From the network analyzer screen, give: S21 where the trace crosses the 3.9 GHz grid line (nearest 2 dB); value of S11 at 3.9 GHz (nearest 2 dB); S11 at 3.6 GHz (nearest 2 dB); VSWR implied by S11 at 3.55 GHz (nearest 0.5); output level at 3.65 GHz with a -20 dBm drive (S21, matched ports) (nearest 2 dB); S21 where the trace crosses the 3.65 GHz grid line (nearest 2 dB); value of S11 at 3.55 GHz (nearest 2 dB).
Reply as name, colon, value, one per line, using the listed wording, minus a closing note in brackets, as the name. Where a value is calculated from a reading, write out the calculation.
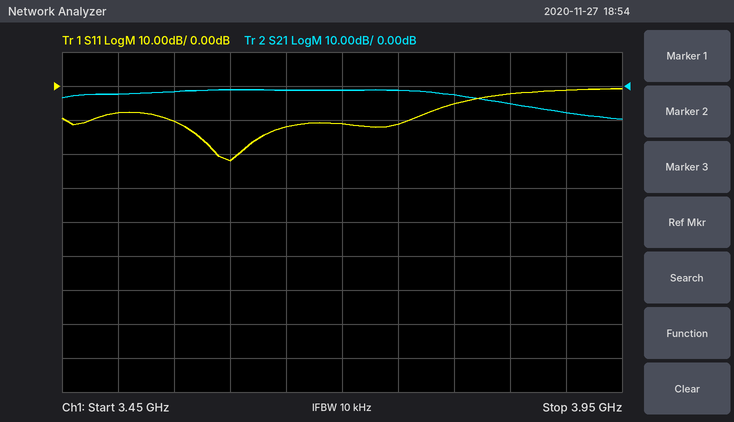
S21 where the trace crosses the 3.9 GHz grid line: -8 dB
value of S11 at 3.9 GHz: -2 dB
S11 at 3.6 GHz: -22 dB
VSWR implied by S11 at 3.55 GHz: |Γ| = 10^(-10/20) = 0.3162; VSWR = (1 + 0.3162)/(1 − 0.3162) ≈ 1.92, so 2.0 to the nearest 0.5
output level at 3.65 GHz with a -20 dBm drive (S21, matched ports): -20 dBm + (-2 dB) = -22 dBm
S21 where the trace crosses the 3.65 GHz grid line: -2 dB
value of S11 at 3.55 GHz: -10 dB
